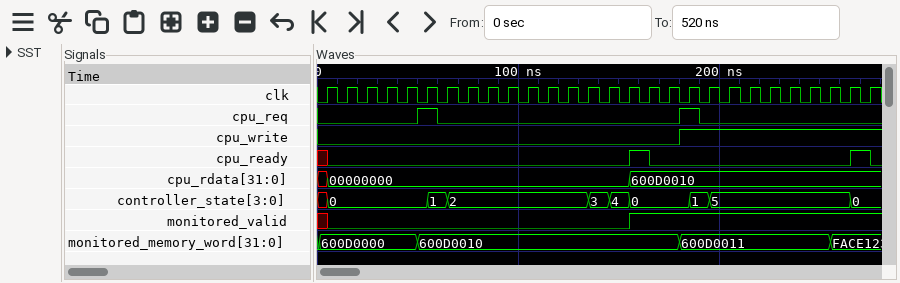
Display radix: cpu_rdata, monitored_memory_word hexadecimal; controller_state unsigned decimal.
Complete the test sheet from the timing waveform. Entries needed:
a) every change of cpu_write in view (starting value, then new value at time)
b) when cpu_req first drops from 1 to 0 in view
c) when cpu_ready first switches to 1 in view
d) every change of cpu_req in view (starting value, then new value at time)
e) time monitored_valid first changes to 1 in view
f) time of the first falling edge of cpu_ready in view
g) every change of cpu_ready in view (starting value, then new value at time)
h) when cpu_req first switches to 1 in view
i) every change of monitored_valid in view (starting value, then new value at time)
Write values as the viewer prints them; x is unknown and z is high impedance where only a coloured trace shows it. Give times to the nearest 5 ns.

0, 1 at 180 ns
60 ns
155 ns
0, 1 at 50 ns, 0 at 60 ns, 1 at 180 ns, 0 at 190 ns
155 ns
165 ns
x, 0 at 5 ns, 1 at 155 ns, 0 at 165 ns, 1 at 265 ns, 0 at 275 ns
50 ns
x, 0 at 5 ns, 1 at 155 ns
